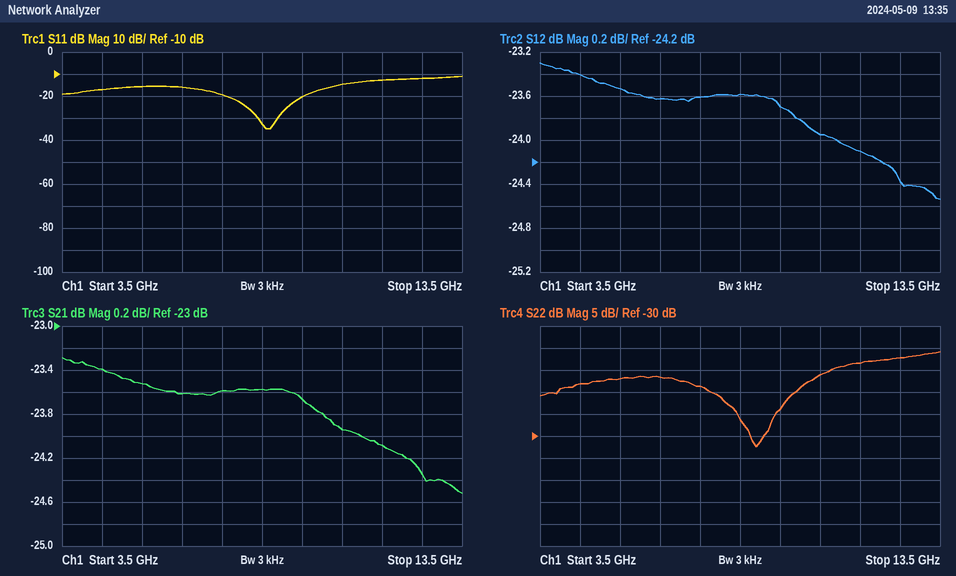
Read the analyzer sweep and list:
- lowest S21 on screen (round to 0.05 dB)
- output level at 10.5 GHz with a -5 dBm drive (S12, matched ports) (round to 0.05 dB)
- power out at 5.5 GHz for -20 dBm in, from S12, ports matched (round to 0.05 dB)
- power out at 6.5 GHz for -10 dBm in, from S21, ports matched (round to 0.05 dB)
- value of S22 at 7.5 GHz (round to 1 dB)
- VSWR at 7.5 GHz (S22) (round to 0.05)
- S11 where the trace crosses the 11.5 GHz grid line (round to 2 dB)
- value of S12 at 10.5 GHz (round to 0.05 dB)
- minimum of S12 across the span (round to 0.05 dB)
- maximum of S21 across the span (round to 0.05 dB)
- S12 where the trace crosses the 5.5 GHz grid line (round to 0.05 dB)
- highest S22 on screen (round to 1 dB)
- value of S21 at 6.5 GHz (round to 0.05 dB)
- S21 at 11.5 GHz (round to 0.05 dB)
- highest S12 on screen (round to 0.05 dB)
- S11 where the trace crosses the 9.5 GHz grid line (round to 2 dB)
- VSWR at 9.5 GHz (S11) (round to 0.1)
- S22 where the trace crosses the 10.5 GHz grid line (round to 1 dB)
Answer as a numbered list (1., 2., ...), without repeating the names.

1. -24.50 dB
2. -28.95 dBm
3. -43.55 dBm
4. -33.60 dBm
5. -19 dB
6. 1.25
7. -12 dB
8. -23.95 dB
9. -24.55 dB
10. -23.30 dB
11. -23.55 dB
12. -11 dB
13. -23.60 dB
14. -24.10 dB
15. -23.30 dB
16. -20 dB
17. 1.2
18. -16 dB
